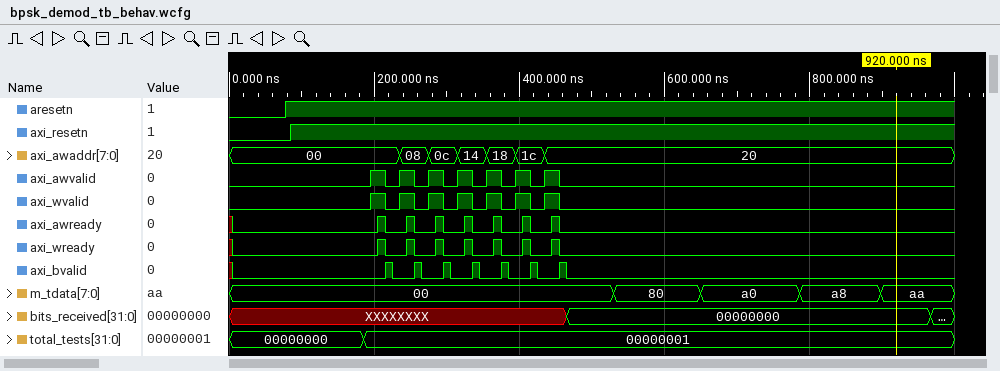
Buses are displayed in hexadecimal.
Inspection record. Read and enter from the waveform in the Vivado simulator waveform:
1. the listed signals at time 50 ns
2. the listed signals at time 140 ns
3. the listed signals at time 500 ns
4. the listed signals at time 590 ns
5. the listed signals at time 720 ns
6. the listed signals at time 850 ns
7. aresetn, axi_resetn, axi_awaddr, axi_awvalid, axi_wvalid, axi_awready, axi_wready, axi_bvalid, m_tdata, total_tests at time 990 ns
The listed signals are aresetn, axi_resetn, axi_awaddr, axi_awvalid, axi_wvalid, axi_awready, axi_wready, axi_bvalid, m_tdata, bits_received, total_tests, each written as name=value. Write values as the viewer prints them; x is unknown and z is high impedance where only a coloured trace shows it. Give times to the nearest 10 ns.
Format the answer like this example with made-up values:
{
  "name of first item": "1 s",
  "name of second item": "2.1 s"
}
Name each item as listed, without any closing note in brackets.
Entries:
{
  "the listed signals at time 50 ns": "aresetn=0, axi_resetn=0, axi_awaddr=00, axi_awvalid=0, axi_wvalid=0, axi_awready=0, axi_wready=0, axi_bvalid=0, m_tdata=00, bits_received=XXXXXXXX, total_tests=00000000",
  "the listed signals at time 140 ns": "aresetn=1, axi_resetn=1, axi_awaddr=00, axi_awvalid=0, axi_wvalid=0, axi_awready=0, axi_wready=0, axi_bvalid=0, m_tdata=00, bits_received=XXXXXXXX, total_tests=00000000",
  "the listed signals at time 500 ns": "aresetn=1, axi_resetn=1, axi_awaddr=20, axi_awvalid=0, axi_wvalid=0, axi_awready=0, axi_wready=0, axi_bvalid=0, m_tdata=00, bits_received=00000000, total_tests=00000001",
  "the listed signals at time 590 ns": "aresetn=1, axi_resetn=1, axi_awaddr=20, axi_awvalid=0, axi_wvalid=0, axi_awready=0, axi_wready=0, axi_bvalid=0, m_tdata=80, bits_received=00000000, total_tests=00000001",
  "the listed signals at time 720 ns": "aresetn=1, axi_resetn=1, axi_awaddr=20, axi_awvalid=0, axi_wvalid=0, axi_awready=0, axi_wready=0, axi_bvalid=0, m_tdata=a0, bits_received=00000000, total_tests=00000001",
  "the listed signals at time 850 ns": "aresetn=1, axi_resetn=1, axi_awaddr=20, axi_awvalid=0, axi_wvalid=0, axi_awready=0, axi_wready=0, axi_bvalid=0, m_tdata=a8, bits_received=00000000, total_tests=00000001",
  "aresetn, axi_resetn, axi_awaddr, axi_awvalid, axi_wvalid, axi_awready, axi_wready, axi_bvalid, m_tdata, total_tests at time 990 ns": "aresetn=1, axi_resetn=1, axi_awaddr=20, axi_awvalid=0, axi_wvalid=0, axi_awready=0, axi_wready=0, axi_bvalid=0, m_tdata=aa, total_tests=00000001"
}
